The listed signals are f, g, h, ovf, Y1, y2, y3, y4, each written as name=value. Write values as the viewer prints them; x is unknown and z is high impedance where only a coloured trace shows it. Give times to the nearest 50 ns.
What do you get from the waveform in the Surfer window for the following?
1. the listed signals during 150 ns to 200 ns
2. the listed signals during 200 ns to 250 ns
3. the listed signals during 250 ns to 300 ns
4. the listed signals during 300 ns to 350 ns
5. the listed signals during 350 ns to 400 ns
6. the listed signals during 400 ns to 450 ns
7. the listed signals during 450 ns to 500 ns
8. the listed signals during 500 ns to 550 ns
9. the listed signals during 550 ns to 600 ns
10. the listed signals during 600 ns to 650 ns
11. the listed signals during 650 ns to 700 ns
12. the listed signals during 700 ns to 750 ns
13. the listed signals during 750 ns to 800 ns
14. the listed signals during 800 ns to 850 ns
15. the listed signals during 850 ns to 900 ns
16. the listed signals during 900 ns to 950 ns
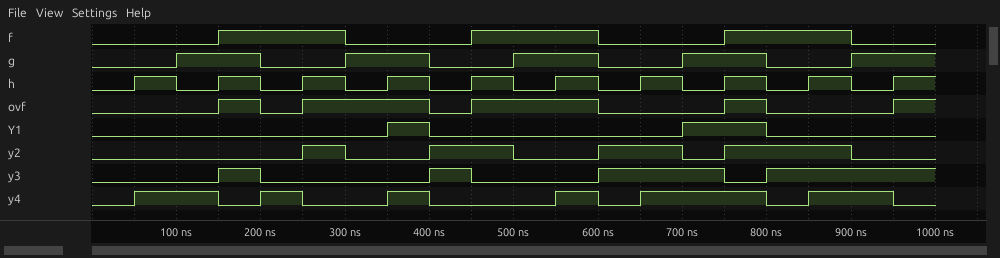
f=1, g=1, h=1, ovf=1, Y1=0, y2=0, y3=1, y4=0
f=1, g=0, h=0, ovf=0, Y1=0, y2=0, y3=0, y4=1
f=1, g=0, h=1, ovf=1, Y1=0, y2=1, y3=0, y4=0
f=0, g=1, h=0, ovf=1, Y1=0, y2=0, y3=0, y4=0
f=0, g=1, h=1, ovf=1, Y1=1, y2=0, y3=0, y4=1
f=0, g=0, h=0, ovf=0, Y1=0, y2=1, y3=1, y4=0
f=1, g=0, h=1, ovf=1, Y1=0, y2=1, y3=0, y4=0
f=1, g=1, h=0, ovf=1, Y1=0, y2=0, y3=0, y4=0
f=1, g=1, h=1, ovf=1, Y1=0, y2=0, y3=0, y4=1
f=0, g=0, h=0, ovf=0, Y1=0, y2=1, y3=1, y4=0
f=0, g=0, h=1, ovf=0, Y1=0, y2=1, y3=1, y4=1
f=0, g=1, h=0, ovf=0, Y1=1, y2=0, y3=1, y4=1
f=1, g=1, h=1, ovf=1, Y1=1, y2=1, y3=0, y4=1
f=1, g=0, h=0, ovf=0, Y1=0, y2=1, y3=1, y4=0
f=1, g=0, h=1, ovf=0, Y1=0, y2=1, y3=1, y4=1
f=0, g=1, h=0, ovf=0, Y1=0, y2=0, y3=1, y4=1
